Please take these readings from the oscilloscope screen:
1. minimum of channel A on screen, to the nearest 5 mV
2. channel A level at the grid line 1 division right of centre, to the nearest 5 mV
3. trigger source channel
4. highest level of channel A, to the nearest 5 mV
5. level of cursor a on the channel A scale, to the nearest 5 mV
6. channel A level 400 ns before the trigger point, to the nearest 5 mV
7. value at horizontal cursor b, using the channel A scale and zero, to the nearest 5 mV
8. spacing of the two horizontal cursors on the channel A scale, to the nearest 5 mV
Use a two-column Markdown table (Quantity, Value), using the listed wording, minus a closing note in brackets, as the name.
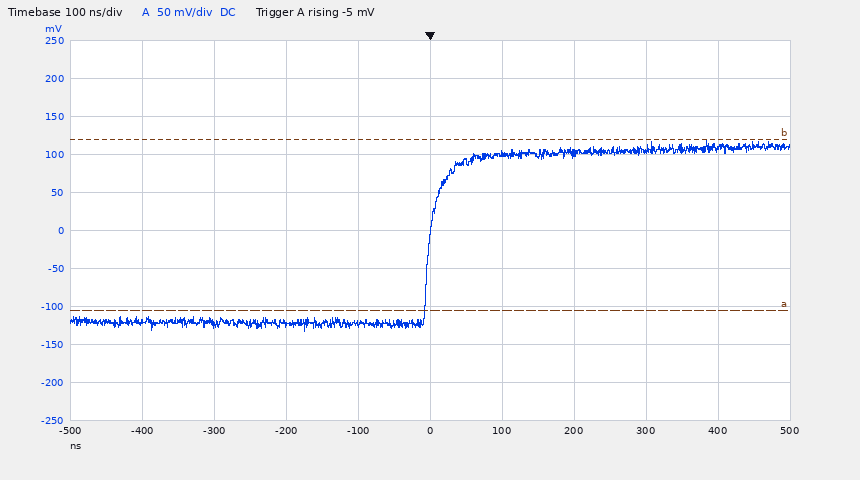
| Quantity | Value |
|---|---|
| minimum of channel A on screen, to the nearest 5 mV | -135 mV |
| channel A level at the grid line 1 division right of centre, to the nearest 5 mV | 100 mV |
| trigger source channel | channel A |
| highest level of channel A, to the nearest 5 mV | 120 mV |
| level of cursor a on the channel A scale, to the nearest 5 mV | -105 mV |
| channel A level 400 ns before the trigger point, to the nearest 5 mV | -120 mV |
| value at horizontal cursor b, using the channel A scale and zero, to the nearest 5 mV | 120 mV |
| spacing of the two horizontal cursors on the channel A scale, to the nearest 5 mV | 225 mV |
